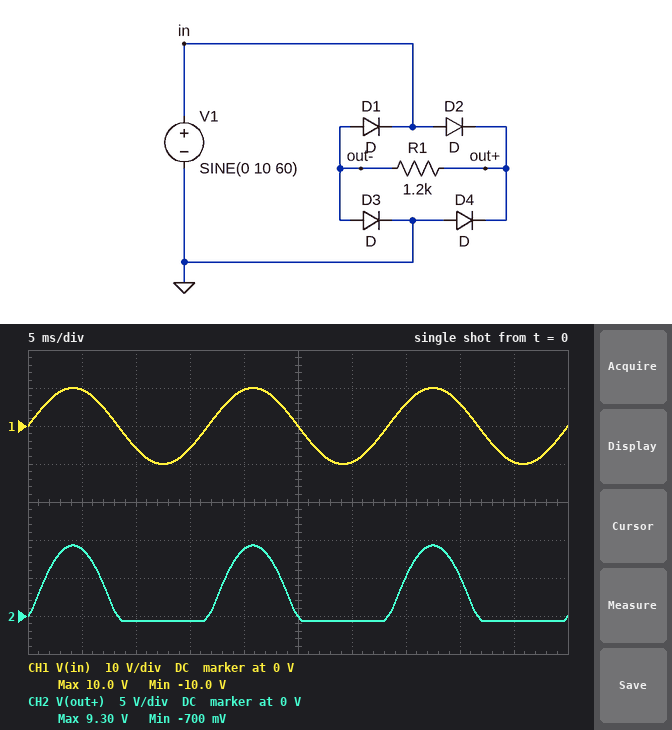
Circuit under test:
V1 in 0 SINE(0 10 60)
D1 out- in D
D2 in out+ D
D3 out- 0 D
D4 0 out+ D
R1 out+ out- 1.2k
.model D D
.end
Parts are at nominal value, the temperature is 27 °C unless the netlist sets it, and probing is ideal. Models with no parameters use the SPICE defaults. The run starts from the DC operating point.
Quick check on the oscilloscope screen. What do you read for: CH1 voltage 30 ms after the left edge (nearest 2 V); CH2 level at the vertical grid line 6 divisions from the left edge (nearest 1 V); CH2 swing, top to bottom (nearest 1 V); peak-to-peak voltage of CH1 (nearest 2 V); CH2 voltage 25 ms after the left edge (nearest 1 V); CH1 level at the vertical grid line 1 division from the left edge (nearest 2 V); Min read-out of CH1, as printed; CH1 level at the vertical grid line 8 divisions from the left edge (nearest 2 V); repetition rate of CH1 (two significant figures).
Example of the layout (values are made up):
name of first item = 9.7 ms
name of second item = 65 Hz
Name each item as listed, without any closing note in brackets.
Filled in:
CH1 voltage 30 ms after the left edge = -10 V
CH2 level at the vertical grid line 6 divisions from the left edge = -1 V
CH2 swing, top to bottom = 10 V
peak-to-peak voltage of CH1 = 20 V
CH2 voltage 25 ms after the left edge = 0 V
CH1 level at the vertical grid line 1 division from the left edge = 10 V
Min read-out of CH1, as printed = -10.0 V
CH1 level at the vertical grid line 8 divisions from the left edge = 6 V
repetition rate of CH1 = 60 Hz
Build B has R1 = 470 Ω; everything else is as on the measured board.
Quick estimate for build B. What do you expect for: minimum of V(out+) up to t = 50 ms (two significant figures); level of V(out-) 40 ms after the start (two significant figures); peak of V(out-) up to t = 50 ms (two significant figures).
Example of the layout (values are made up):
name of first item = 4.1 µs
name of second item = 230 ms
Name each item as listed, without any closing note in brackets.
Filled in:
minimum of V(out+) up to t = 50 ms = -730 mV
level of V(out-) 40 ms after the start = 710 mV
peak of V(out-) up to t = 50 ms = 730 mV
